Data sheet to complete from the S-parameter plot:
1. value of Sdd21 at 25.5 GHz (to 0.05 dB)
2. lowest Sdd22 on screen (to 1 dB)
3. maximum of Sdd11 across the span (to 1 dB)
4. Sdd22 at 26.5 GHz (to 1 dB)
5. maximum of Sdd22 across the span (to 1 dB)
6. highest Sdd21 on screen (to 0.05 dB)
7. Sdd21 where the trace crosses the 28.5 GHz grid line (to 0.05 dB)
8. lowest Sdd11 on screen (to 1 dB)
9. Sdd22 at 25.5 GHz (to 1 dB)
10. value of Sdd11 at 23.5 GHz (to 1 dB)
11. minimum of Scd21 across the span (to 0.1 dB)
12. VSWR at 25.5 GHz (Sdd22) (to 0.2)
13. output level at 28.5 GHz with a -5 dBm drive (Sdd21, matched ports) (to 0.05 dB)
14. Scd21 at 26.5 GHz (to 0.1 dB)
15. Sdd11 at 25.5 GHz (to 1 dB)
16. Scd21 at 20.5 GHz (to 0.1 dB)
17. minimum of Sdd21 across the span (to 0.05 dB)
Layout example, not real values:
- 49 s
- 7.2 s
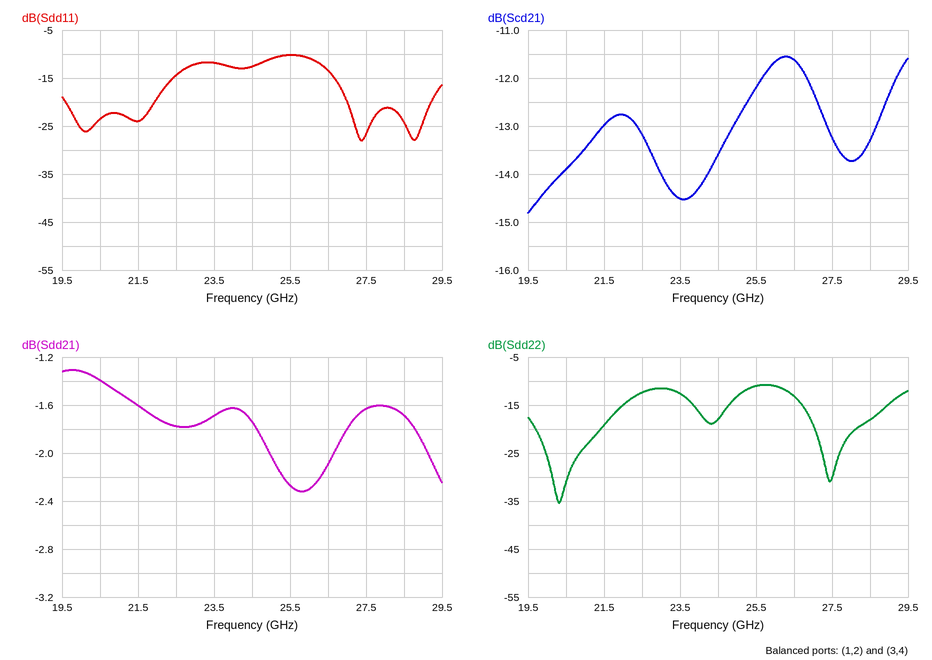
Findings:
- -2.25 dB
- -35 dB
- -10 dB
- -13 dB
- -11 dB
- -1.30 dB
- -1.70 dB
- -28 dB
- -11 dB
- -12 dB
- -14.8 dB
- 1.8
- -6.70 dBm
- -11.6 dB
- -10 dB
- -13.9 dB
- -2.30 dB
